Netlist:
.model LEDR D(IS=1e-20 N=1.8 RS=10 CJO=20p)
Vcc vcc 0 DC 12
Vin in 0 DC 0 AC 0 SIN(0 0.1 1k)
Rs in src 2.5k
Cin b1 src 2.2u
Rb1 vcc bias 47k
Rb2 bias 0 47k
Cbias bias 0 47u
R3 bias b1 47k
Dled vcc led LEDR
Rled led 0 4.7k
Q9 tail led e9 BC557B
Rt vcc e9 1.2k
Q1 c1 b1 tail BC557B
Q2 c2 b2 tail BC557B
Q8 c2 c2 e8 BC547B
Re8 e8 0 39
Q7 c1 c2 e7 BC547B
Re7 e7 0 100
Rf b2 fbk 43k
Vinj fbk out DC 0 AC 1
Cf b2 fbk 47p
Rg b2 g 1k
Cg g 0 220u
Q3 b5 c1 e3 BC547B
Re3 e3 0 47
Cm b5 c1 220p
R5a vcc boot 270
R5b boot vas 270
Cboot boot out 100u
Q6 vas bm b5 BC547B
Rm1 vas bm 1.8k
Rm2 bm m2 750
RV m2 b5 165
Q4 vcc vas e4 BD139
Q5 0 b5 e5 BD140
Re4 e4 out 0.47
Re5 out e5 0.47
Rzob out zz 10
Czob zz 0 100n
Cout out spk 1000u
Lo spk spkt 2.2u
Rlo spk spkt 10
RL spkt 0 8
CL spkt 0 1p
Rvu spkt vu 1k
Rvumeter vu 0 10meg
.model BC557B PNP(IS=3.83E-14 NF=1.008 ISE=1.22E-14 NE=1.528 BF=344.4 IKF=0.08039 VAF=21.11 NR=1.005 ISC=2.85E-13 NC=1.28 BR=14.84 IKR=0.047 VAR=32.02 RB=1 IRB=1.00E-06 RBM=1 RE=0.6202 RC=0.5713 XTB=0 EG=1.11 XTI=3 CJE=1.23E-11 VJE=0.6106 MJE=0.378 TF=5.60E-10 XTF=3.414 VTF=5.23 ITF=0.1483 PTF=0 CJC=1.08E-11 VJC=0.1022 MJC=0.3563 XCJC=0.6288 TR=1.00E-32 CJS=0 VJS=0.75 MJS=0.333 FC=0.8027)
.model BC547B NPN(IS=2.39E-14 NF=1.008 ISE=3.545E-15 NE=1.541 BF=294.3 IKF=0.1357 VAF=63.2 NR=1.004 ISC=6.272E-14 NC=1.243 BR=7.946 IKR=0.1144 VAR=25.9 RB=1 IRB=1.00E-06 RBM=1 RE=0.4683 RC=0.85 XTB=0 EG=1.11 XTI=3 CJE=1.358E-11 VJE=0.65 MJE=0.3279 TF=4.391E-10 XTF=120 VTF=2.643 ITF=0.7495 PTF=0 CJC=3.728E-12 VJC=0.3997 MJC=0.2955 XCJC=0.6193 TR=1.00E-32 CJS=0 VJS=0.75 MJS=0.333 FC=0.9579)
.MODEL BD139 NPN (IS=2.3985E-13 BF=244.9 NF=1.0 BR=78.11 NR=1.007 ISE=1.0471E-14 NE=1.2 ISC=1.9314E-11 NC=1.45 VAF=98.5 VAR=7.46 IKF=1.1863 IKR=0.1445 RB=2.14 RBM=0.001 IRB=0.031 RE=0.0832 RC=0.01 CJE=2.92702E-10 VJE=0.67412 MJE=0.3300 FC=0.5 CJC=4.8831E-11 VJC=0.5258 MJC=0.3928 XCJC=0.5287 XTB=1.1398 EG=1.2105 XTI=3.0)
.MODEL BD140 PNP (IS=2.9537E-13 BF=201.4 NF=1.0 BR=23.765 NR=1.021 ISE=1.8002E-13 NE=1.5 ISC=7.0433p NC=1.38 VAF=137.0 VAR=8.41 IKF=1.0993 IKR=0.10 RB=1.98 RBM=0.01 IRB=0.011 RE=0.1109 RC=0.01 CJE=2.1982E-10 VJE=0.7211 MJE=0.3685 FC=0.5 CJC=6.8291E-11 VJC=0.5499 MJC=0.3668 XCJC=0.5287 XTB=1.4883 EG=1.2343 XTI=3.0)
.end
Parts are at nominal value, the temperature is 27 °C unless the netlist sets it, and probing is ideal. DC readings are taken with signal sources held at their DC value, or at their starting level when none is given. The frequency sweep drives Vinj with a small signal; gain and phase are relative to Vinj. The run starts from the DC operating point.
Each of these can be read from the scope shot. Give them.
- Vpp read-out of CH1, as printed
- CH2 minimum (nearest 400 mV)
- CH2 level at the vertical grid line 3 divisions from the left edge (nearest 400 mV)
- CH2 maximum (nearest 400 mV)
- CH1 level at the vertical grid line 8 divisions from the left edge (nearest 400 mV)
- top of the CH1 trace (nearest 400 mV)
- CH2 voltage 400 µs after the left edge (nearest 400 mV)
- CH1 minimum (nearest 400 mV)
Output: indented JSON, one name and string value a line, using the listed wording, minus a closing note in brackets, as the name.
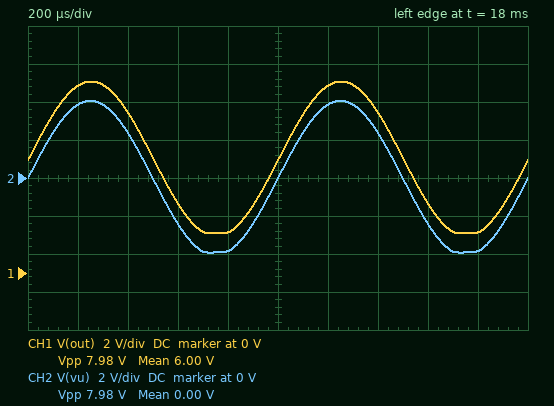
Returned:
{
  "Vpp read-out of CH1, as printed": "7.98 V",
  "CH2 minimum": "-4.0 V",
  "CH2 level at the vertical grid line 3 divisions from the left edge": "-2.4 V",
  "CH2 maximum": "4.0 V",
  "CH1 level at the vertical grid line 8 divisions from the left edge": "3.6 V",
  "top of the CH1 trace": "10.0 V",
  "CH2 voltage 400 µs after the left edge": "2.4 V",
  "CH1 minimum": "2.0 V"
}
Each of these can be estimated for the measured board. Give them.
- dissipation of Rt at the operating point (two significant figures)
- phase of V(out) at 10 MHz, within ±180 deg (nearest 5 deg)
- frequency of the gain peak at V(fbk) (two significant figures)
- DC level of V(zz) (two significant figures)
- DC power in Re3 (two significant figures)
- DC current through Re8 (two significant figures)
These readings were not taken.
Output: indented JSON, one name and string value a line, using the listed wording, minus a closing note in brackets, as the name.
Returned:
{
  "dissipation of Rt at the operating point": "1.3 mW",
  "phase of V(out) at 10 MHz, within ±180 deg": "5 deg",
  "frequency of the gain peak at V(fbk)": "6.0 MHz",
  "DC level of V(zz)": "6.0 V",
  "DC power in Re3": "4.5 mW",
  "DC current through Re8": "630 µA"
}
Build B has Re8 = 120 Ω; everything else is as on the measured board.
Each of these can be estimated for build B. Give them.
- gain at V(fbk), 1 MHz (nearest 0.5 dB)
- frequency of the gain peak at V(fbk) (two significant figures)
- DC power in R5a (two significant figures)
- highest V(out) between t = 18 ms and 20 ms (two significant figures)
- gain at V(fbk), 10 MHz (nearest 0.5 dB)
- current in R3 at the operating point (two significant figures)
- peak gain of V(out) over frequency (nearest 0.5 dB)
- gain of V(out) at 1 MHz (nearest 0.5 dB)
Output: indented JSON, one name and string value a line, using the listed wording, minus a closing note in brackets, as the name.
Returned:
{
  "gain at V(fbk), 1 MHz": "-11.0 dB",
  "frequency of the gain peak at V(fbk)": "6.8 MHz",
  "DC power in R5a": "22 mW",
  "highest V(out) between t = 18 ms and 20 ms": "10 V",
  "gain at V(fbk), 10 MHz": "3.5 dB",
  "current in R3 at the operating point": "1.4 µA",
  "peak gain of V(out) over frequency": "1.5 dB",
  "gain of V(out) at 1 MHz": "-2.0 dB"
}
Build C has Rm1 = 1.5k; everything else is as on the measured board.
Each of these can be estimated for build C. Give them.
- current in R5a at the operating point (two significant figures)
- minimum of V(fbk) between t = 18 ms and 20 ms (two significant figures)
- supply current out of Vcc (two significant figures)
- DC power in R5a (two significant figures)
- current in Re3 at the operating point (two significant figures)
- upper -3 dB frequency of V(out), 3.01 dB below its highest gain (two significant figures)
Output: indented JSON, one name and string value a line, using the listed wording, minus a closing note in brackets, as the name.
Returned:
{
  "current in R5a at the operating point": "9.4 mA",
  "minimum of V(fbk) between t = 18 ms and 20 ms": "2.0 V",
  "supply current out of Vcc": "360 mA",
  "DC power in R5a": "24 mW",
  "current in Re3 at the operating point": "9.7 mA",
  "upper -3 dB frequency of V(out), 3.01 dB below its highest gain": "5.5 MHz"
}
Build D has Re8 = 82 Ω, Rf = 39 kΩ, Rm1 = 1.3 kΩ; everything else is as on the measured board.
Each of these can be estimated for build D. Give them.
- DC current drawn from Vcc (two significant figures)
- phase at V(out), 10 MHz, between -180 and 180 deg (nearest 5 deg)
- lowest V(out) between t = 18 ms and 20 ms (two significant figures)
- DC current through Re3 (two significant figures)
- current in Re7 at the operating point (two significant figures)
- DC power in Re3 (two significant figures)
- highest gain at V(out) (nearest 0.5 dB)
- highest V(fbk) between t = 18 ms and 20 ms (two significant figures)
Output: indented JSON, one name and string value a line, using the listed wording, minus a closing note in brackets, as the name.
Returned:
{
  "DC current drawn from Vcc": "250 mA",
  "phase at V(out), 10 MHz, between -180 and 180 deg": "0 deg",
  "lowest V(out) between t = 18 ms and 20 ms": "2.3 V",
  "DC current through Re3": "9.7 mA",
  "current in Re7 at the operating point": "470 µA",
  "DC power in Re3": "4.4 mW",
  "highest gain at V(out)": "0 dB",
  "highest V(fbk) between t = 18 ms and 20 ms": "9.8 V"
}
